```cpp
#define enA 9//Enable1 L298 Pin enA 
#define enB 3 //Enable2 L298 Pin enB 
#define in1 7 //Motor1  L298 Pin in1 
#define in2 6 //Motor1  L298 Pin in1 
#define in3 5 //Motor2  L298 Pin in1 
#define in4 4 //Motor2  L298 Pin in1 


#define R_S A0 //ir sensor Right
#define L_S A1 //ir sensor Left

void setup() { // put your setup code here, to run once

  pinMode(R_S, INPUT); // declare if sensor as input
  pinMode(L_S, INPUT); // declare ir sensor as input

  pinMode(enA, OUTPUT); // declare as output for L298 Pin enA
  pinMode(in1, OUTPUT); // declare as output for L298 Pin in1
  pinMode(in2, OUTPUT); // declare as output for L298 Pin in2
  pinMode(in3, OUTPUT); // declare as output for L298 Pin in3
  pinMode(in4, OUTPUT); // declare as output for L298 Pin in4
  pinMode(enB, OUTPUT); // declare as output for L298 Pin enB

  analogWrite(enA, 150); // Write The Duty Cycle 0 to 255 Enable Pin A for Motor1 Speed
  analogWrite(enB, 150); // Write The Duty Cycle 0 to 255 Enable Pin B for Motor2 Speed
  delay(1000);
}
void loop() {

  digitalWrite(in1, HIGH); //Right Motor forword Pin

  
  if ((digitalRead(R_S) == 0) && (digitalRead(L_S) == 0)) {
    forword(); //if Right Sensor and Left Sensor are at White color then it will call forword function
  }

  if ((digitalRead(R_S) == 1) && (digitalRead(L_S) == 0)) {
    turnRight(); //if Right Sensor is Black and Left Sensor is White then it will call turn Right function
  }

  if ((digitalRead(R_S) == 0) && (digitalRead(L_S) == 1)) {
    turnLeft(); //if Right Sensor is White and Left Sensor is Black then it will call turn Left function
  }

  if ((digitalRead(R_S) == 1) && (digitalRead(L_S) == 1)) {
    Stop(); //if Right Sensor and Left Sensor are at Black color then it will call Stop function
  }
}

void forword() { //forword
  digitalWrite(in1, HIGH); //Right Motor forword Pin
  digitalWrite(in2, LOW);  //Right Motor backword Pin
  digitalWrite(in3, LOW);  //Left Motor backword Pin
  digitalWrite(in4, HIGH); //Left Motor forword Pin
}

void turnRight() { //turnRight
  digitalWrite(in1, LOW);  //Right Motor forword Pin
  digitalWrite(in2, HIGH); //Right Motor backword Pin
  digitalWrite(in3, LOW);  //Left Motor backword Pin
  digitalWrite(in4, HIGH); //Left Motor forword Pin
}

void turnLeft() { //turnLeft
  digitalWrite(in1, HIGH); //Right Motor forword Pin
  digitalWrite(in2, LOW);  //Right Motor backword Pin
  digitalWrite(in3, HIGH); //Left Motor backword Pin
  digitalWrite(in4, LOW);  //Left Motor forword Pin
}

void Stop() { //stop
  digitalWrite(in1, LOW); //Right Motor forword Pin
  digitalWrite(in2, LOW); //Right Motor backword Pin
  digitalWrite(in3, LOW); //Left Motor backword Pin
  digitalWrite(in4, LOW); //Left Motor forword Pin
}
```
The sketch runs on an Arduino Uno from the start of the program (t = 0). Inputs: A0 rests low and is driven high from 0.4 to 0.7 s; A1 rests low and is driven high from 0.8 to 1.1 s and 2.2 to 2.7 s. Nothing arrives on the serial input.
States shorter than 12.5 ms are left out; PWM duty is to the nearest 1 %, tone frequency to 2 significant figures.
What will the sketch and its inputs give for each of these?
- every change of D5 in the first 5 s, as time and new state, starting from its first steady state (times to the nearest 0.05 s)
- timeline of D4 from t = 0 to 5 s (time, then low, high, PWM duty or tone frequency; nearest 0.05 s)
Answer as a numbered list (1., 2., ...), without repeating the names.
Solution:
1. 0 s low; 1 s high; 1.1 s low; 2.2 s high; 2.7 s low
2. 0 s low; 1.1 s high; 2.2 s low; 2.7 s high
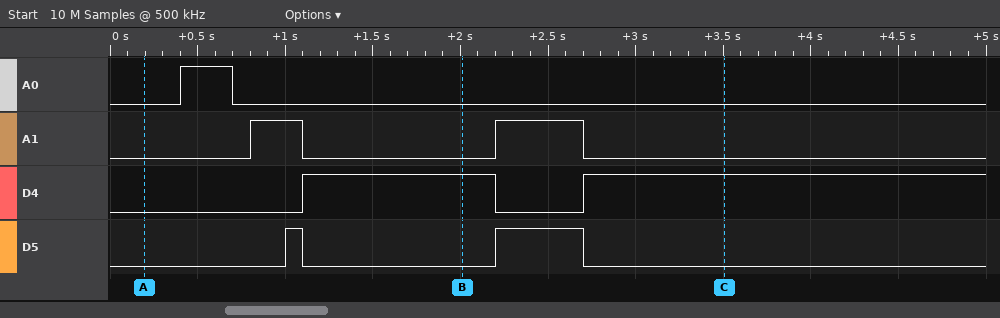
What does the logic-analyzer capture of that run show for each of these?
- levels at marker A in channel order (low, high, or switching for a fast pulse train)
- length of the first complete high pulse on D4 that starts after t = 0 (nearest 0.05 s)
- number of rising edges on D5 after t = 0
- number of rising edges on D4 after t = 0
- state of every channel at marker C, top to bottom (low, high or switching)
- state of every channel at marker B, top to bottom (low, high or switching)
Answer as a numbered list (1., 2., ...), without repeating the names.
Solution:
1. A0 low, A1 low, D4 low, D5 low
2. 1.10 s
3. 2
4. 2
5. A0 low, A1 low, D4 high, D5 low
6. A0 low, A1 low, D4 high, D5 low
